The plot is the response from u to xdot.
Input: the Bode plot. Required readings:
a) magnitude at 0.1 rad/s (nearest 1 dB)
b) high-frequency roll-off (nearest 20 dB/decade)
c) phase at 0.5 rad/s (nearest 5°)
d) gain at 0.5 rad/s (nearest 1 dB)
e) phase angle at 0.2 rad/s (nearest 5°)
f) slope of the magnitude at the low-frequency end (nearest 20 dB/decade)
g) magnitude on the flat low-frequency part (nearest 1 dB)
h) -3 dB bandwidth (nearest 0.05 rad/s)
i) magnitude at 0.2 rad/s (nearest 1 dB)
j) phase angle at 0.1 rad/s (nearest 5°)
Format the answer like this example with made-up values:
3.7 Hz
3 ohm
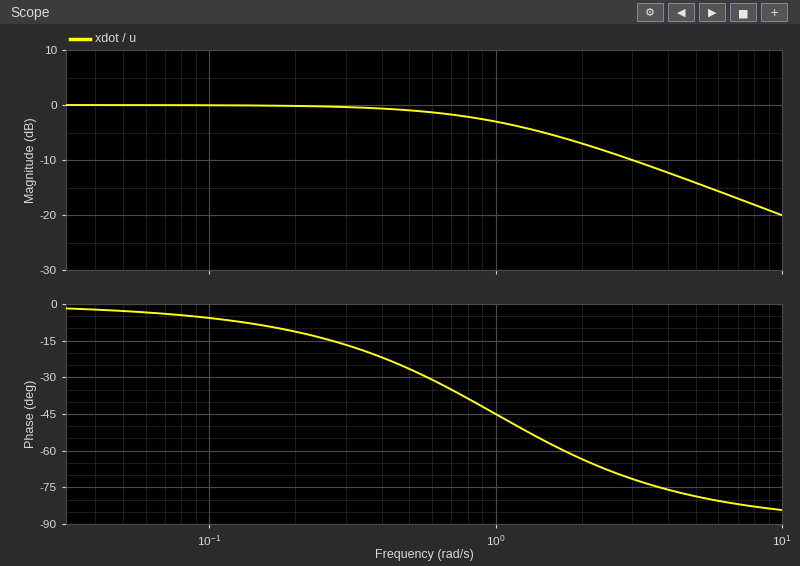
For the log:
0 dB
-20 dB/decade
-25°
-1 dB
-10°
0 dB/decade
0 dB
1.00 rad/s
0 dB
-5°
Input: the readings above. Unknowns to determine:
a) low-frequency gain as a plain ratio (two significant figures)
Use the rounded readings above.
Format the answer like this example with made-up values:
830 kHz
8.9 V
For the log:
1.0
